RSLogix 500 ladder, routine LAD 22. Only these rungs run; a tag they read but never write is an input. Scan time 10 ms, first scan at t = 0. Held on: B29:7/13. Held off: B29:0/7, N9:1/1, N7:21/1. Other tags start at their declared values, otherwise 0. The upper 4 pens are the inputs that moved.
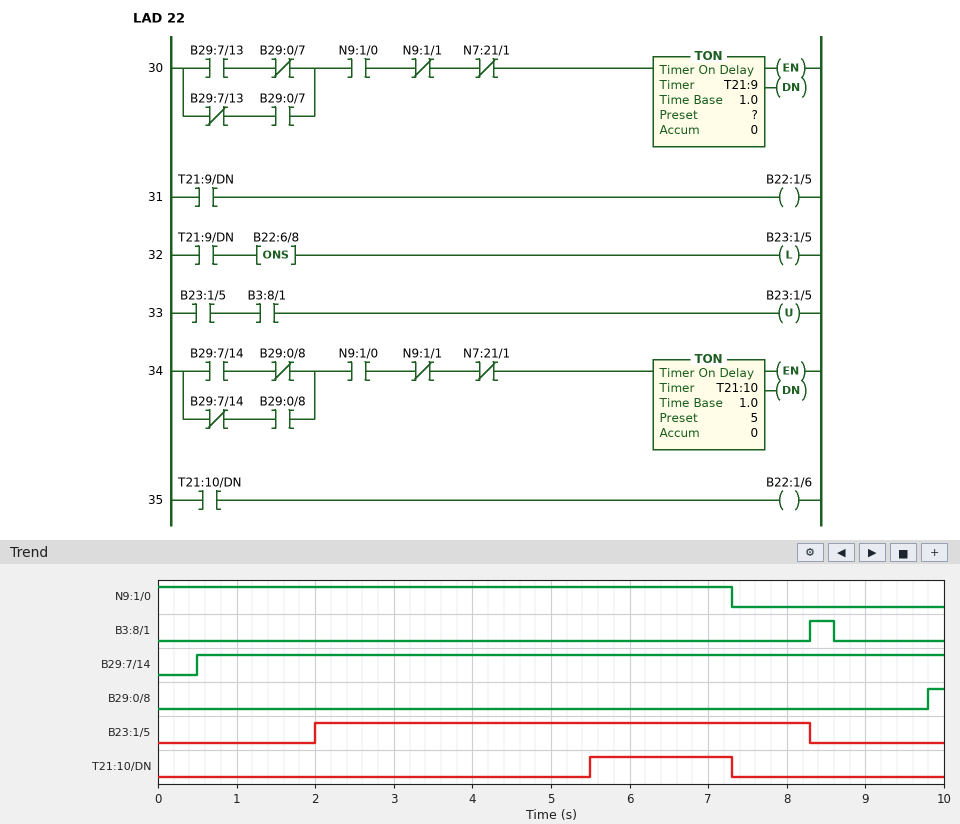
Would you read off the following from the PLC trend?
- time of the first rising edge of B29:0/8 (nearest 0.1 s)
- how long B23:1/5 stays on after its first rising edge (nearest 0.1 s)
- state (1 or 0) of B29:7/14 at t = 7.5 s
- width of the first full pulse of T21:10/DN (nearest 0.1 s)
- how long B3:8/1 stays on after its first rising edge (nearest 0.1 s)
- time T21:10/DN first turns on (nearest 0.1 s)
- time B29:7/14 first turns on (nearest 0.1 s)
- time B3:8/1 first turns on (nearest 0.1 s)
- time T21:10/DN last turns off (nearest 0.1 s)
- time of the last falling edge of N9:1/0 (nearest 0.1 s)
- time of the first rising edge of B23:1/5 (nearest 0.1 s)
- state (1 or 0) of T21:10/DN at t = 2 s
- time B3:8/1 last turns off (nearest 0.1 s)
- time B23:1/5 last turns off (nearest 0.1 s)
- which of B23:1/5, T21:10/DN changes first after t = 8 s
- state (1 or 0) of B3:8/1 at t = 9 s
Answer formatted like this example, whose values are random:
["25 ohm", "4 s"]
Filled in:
["9.8 s", "6.3 s", "1", "1.8 s", "0.3 s", "5.5 s", "0.5 s", "8.3 s", "7.3 s", "7.3 s", "2.0 s", "0", "8.6 s", "8.3 s", "B23:1/5", "0"]
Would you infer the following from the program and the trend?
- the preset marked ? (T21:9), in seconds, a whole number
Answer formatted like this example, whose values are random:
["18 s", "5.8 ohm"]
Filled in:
["2 s"]
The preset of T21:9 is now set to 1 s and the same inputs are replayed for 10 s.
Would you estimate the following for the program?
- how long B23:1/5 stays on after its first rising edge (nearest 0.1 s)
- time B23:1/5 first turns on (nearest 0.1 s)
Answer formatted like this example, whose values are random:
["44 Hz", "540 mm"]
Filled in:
["7.3 s", "1.0 s"]
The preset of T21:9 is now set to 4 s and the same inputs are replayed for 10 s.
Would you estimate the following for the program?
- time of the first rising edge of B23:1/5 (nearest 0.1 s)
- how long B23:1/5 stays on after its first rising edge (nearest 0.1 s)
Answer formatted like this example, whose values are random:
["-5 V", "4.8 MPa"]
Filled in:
["4.0 s", "4.3 s"]
